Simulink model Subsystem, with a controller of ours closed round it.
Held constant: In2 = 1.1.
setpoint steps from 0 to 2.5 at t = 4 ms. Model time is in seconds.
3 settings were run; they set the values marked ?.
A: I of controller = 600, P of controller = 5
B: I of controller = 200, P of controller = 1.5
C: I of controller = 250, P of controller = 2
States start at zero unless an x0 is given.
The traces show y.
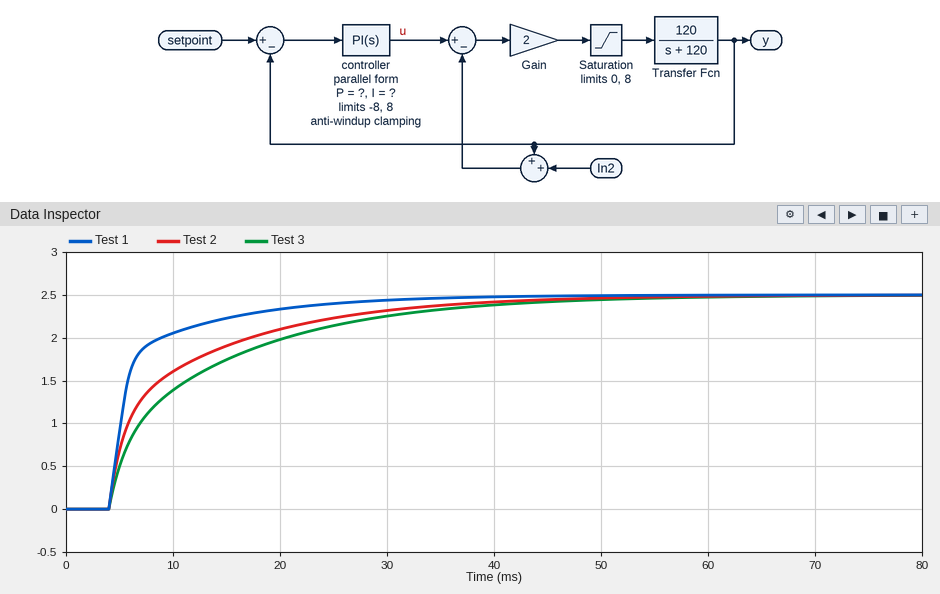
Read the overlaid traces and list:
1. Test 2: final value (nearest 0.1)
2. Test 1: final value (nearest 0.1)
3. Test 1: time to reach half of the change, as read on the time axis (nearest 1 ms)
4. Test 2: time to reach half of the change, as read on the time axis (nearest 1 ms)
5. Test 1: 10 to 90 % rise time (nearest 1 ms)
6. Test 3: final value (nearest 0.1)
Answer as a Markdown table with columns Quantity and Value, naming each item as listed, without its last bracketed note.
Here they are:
| Quantity | Value |
|---|---|
| Test 2: final value | 2.5 |
| Test 1: final value | 2.5 |
| Test 1: time to reach half of the change, as read on the time axis | 5 ms |
| Test 2: time to reach half of the change, as read on the time axis | 7 ms |
| Test 1: 10 to 90 % rise time | 12 ms |
| Test 3: final value | 2.5 |
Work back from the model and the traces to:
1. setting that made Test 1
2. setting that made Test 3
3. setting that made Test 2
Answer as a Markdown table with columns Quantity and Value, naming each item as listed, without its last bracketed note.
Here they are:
| Quantity | Value |
|---|---|
| setting that made Test 1 | A |
| setting that made Test 3 | B |
| setting that made Test 2 | C |
